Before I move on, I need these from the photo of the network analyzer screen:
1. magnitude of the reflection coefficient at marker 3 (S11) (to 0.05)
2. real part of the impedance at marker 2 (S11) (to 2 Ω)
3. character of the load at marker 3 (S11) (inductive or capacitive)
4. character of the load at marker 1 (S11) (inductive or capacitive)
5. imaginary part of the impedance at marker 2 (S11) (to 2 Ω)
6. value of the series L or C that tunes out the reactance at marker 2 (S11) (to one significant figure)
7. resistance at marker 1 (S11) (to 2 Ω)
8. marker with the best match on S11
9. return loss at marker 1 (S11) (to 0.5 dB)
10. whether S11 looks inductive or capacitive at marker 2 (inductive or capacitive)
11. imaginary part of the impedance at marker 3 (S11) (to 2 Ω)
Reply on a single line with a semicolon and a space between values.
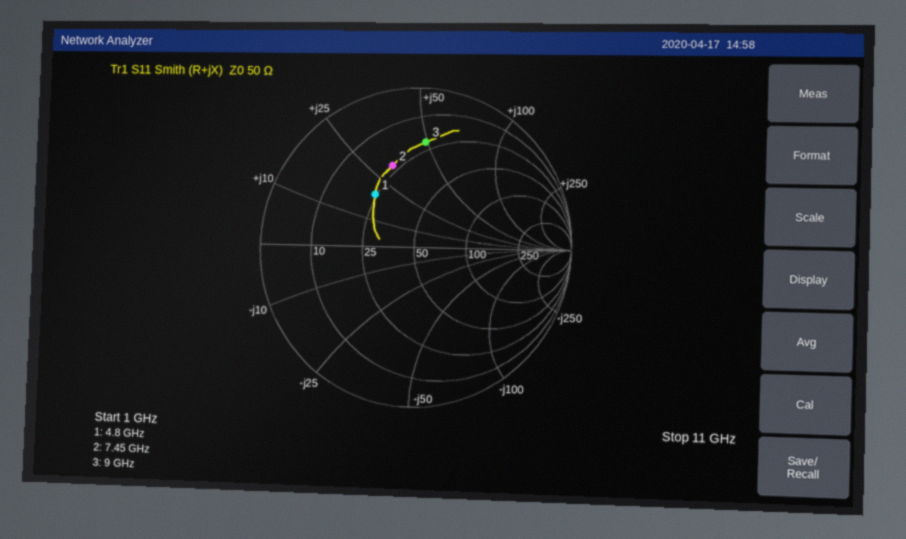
0.65; 22 Ω; inductive; inductive; +32 Ω; 700 fF; 24 Ω; marker 1; 7.5 dB; inductive; +50 Ω
